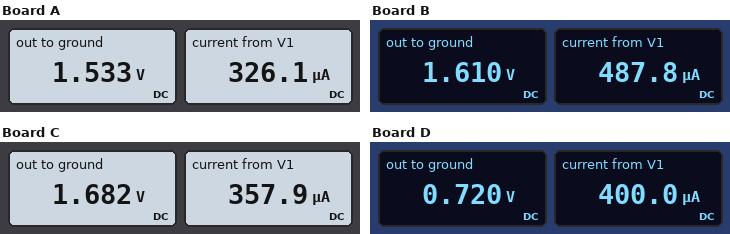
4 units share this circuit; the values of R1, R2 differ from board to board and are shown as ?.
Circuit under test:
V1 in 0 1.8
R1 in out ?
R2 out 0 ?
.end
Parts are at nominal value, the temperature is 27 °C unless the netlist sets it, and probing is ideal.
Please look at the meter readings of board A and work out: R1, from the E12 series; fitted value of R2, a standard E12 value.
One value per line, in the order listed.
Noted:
820 Ω
4.7 kΩ
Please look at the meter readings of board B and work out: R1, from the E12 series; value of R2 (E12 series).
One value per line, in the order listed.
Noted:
390 Ω
3.3 kΩ
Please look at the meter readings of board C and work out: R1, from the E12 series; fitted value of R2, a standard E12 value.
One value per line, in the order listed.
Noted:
330 Ω
4.7 kΩ
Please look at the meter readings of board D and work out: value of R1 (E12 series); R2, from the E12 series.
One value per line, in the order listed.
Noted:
2.7 kΩ
1.8 kΩ
